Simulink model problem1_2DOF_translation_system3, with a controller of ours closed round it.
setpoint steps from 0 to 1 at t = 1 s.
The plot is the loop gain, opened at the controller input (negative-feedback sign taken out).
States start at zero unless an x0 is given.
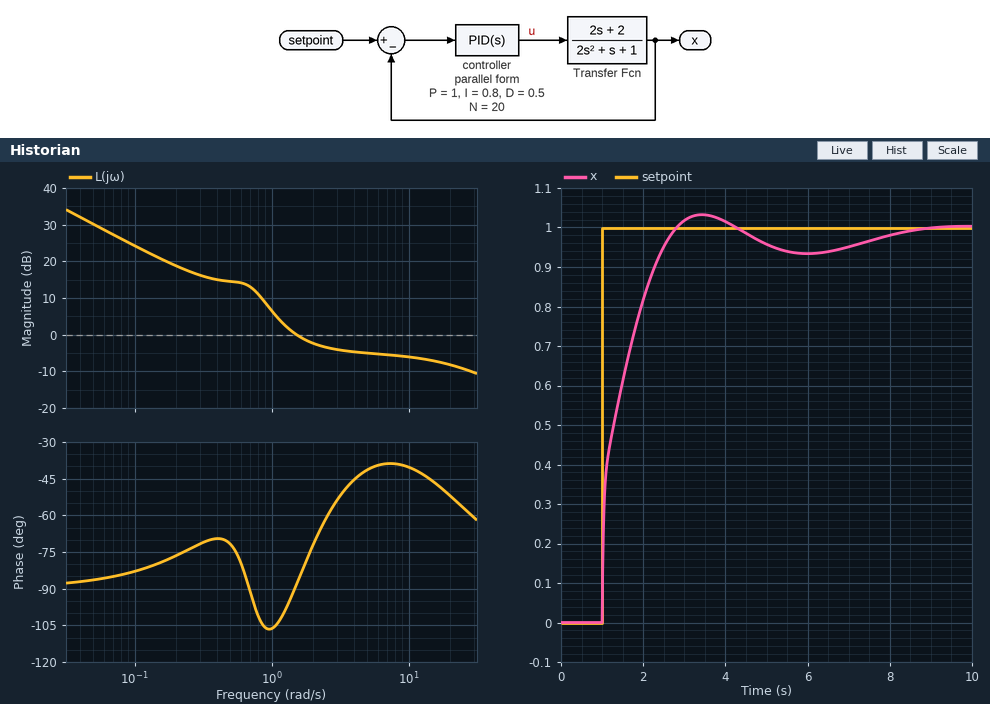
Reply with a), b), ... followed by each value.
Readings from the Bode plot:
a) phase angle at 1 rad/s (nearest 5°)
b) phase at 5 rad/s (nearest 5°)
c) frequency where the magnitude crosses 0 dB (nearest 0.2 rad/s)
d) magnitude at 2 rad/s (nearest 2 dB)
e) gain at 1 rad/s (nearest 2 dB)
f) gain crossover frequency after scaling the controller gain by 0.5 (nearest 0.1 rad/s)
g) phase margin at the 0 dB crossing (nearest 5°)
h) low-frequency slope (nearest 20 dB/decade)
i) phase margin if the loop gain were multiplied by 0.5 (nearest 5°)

a) -105°
b) -40°
c) 1.6 rad/s
d) -2 dB
e) 6 dB
f) 1.0 rad/s
g) 90°
h) -20 dB/decade
i) 75°
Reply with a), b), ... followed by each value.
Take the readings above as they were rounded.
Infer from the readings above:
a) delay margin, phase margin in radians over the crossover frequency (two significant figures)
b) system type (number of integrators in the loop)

a) 0.98 s
b) 1
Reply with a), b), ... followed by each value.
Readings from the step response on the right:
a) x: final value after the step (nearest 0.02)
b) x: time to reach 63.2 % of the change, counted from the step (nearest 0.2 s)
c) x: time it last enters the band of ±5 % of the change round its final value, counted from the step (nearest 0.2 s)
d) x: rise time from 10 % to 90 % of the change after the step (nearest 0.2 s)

a) 1.00
b) 0.6 s
c) 6.0 s
d) 1.2 s
